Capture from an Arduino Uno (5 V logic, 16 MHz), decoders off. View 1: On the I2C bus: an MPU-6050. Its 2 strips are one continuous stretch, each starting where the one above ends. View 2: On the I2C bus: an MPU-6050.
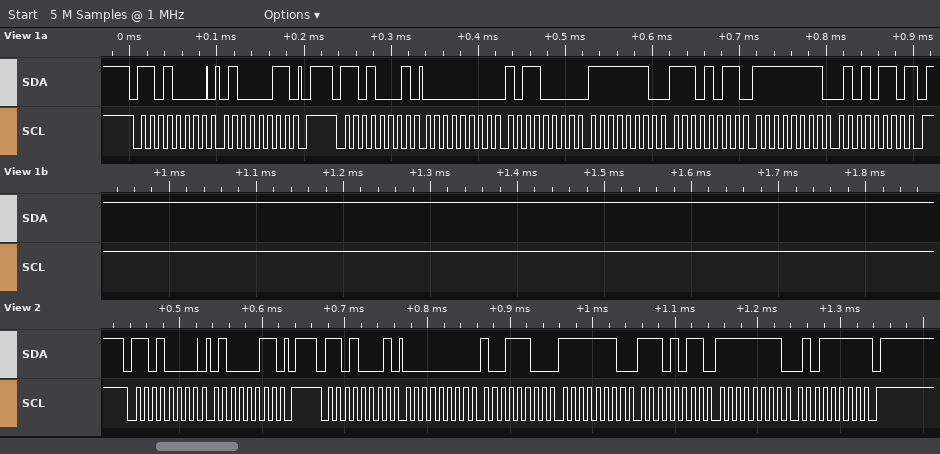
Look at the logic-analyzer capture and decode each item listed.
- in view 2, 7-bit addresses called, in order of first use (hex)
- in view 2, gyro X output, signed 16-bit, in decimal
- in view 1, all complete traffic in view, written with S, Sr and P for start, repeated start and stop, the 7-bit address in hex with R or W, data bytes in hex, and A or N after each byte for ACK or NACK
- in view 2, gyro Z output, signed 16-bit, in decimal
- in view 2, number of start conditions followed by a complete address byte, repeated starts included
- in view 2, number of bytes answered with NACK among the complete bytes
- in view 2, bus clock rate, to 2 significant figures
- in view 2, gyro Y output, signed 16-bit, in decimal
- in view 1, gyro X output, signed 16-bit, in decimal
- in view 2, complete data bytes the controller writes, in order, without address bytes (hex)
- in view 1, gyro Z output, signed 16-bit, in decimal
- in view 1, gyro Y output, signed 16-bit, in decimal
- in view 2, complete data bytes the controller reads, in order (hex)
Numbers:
0x68
156
S 68W A 43 A P S 68R A 00 A B0 A FE A EB A FF A 56 N P
-161
2
1
100 kHz
-277
176
43
-170
-277
00 9C FE EB FF 5F
